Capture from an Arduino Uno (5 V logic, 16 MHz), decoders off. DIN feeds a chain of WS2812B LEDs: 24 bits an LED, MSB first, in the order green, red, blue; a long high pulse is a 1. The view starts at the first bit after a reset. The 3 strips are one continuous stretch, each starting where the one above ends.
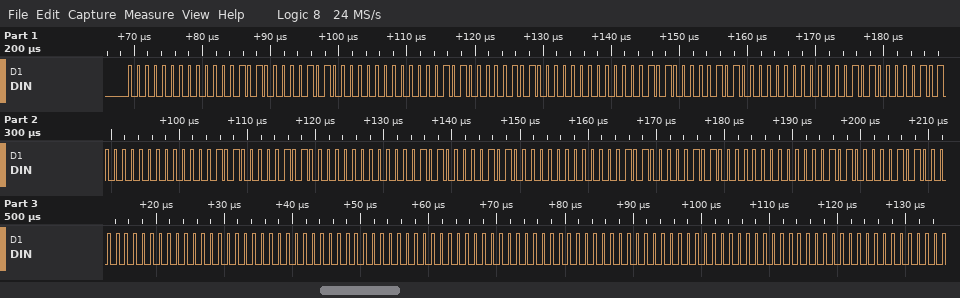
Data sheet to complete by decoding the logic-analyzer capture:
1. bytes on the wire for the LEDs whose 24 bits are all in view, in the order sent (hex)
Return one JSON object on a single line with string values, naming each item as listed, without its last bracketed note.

{"bytes on the wire for the LEDs whose 24 bits are all in view, in the order sent": "00 05 05 00 05 05 00 05 05 00 05 05 00 05 05 00 05 05 00 05 05 00 05 05 00 00 00 00 00 00 00 00 00 00 00 00"}
